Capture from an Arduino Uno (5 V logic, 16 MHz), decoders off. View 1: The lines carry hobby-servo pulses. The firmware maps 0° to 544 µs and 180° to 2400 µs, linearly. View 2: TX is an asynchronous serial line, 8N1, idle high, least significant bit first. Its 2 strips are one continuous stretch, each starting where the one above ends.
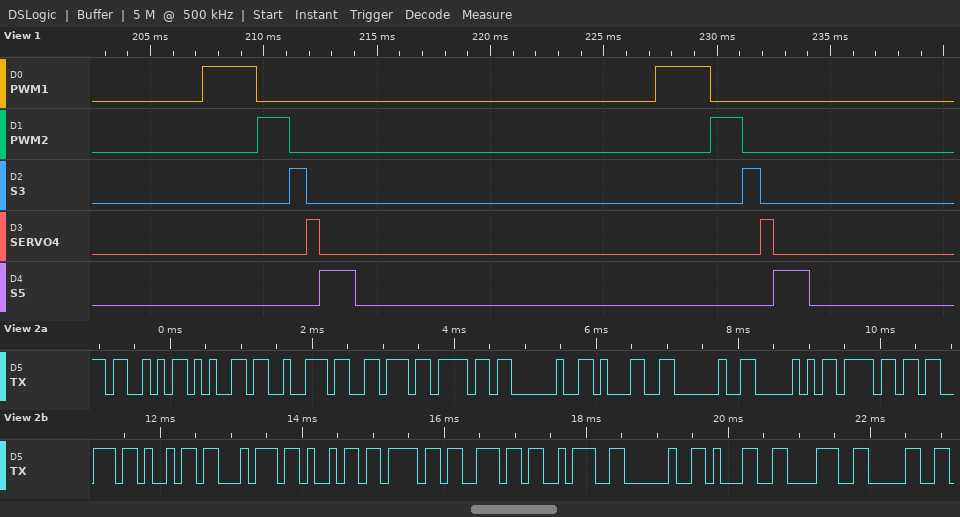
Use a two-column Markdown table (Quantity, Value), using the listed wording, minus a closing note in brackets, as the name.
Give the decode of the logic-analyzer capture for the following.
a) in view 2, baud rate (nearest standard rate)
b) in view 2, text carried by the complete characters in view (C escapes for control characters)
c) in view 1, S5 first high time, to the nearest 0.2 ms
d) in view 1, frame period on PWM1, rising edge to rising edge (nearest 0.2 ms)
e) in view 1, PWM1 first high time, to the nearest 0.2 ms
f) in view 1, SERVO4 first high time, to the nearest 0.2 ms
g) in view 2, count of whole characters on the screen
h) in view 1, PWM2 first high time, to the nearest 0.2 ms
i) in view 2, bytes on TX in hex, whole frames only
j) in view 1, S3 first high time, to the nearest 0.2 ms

| Quantity | Value |
|---|---|
| in view 2, baud rate | 9600 baud |
| in view 2, text carried by the complete characters in view | "Servo 1 Position: 180" |
| in view 1, S5 first high time, to the nearest 0.2 ms | 1.6 ms |
| in view 1, frame period on PWM1, rising edge to rising edge | 20.0 ms |
| in view 1, PWM1 first high time, to the nearest 0.2 ms | 2.4 ms |
| in view 1, SERVO4 first high time, to the nearest 0.2 ms | 0.6 ms |
| in view 2, count of whole characters on the screen | 21 |
| in view 1, PWM2 first high time, to the nearest 0.2 ms | 1.4 ms |
| in view 2, bytes on TX in hex, whole frames only | 0x53 0x65 0x72 0x76 0x6F 0x20 0x31 0x20 0x50 0x6F 0x73 0x69 0x74 0x69 0x6F 0x6E 0x3A 0x20 0x31 0x38 0x30 |
| in view 1, S3 first high time, to the nearest 0.2 ms | 0.8 ms |
